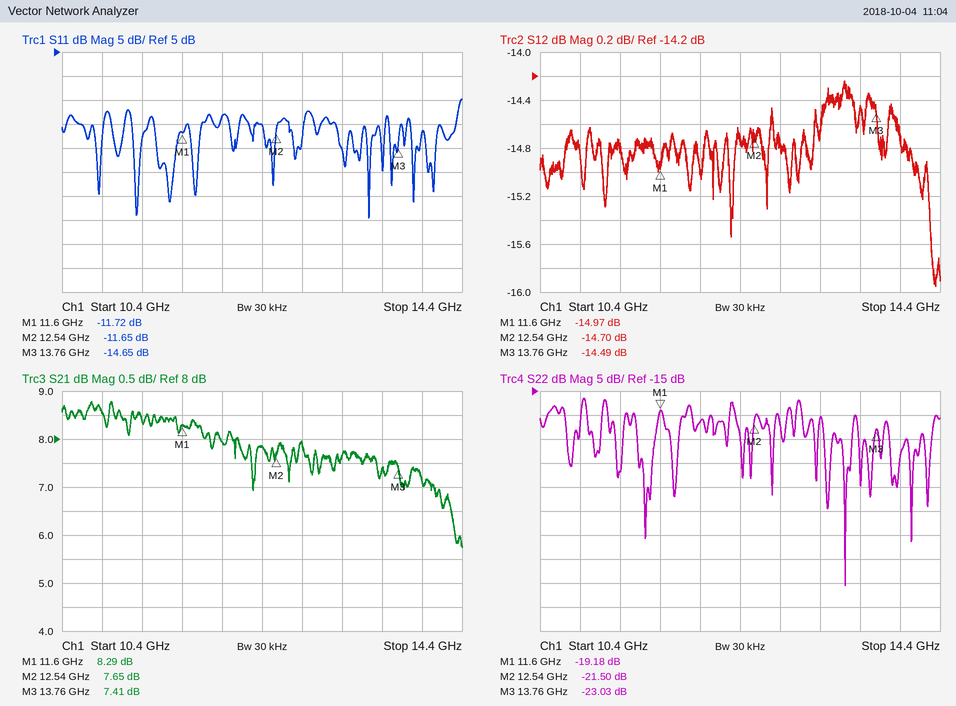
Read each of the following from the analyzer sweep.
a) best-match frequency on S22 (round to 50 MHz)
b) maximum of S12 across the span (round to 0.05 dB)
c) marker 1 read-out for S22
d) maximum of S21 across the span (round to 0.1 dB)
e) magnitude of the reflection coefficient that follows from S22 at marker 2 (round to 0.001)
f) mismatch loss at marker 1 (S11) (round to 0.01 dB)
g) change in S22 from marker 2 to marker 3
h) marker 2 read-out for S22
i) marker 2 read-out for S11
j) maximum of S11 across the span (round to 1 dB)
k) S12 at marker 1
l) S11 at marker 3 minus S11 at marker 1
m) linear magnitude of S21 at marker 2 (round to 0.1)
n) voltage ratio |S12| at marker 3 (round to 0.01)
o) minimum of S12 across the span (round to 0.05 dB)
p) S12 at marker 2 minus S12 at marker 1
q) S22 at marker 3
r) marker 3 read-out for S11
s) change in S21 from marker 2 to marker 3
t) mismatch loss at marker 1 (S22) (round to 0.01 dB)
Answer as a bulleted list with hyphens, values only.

- 13.45 GHz
- -14.25 dB
- -19.18 dB
- 8.8 dB
- 0.084
- 0.30 dB
- -1.53 dB
- -21.50 dB
- -11.65 dB
- -5 dB
- -14.97 dB
- -2.93 dB
- 2.4
- 0.19
- -15.95 dB
- 0.27 dB
- -23.03 dB
- -14.65 dB
- -0.24 dB
- 0.05 dB
